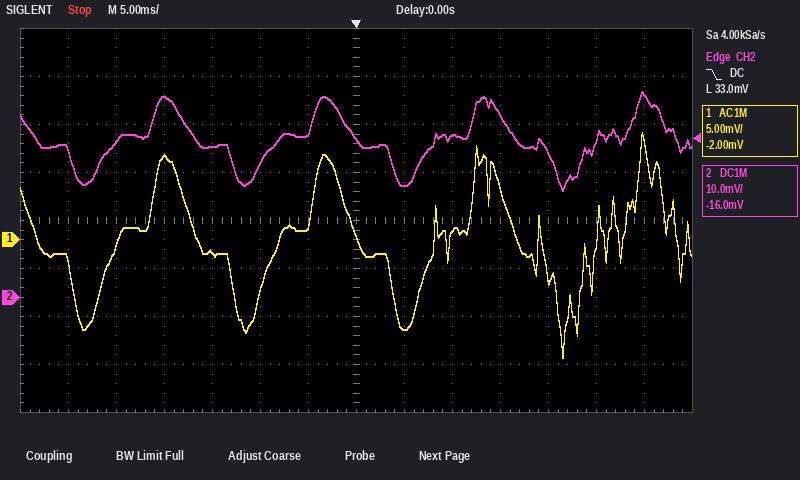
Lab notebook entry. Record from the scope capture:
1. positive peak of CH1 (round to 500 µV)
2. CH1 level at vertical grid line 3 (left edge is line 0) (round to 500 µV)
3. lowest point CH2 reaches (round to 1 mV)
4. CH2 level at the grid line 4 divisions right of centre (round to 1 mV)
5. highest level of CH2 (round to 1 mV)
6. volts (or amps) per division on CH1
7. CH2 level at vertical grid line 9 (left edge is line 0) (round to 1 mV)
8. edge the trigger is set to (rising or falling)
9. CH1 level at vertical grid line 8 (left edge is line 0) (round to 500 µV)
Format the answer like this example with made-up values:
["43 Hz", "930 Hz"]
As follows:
["11.0 mV", "8.5 mV", "22 mV", "30 mV", "43 mV", "5 mV", "34 mV", "falling", "-9.5 mV"]
